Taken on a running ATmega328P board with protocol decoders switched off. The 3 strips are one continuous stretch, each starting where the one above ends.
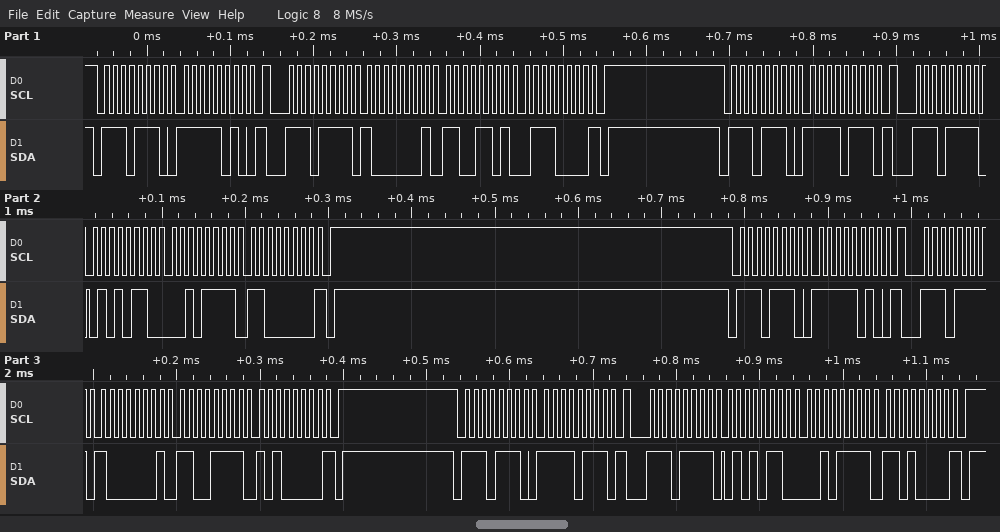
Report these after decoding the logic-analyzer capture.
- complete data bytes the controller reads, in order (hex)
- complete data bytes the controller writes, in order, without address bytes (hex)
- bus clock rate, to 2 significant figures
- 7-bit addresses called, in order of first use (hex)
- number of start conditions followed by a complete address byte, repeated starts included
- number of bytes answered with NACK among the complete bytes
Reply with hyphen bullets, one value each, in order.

- 81 CD 70 56 2F C0 81 CF A0 56 2F D0
- FA F7 FA F7
- 100 kHz
- 0x77
- 8
- 4
